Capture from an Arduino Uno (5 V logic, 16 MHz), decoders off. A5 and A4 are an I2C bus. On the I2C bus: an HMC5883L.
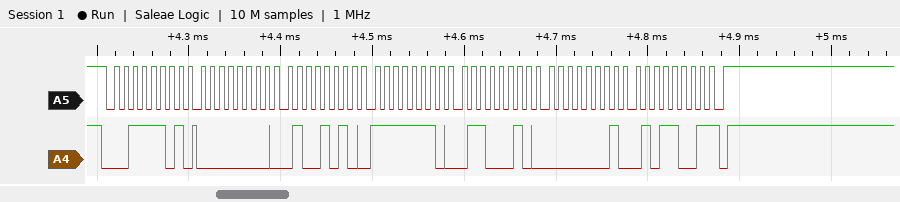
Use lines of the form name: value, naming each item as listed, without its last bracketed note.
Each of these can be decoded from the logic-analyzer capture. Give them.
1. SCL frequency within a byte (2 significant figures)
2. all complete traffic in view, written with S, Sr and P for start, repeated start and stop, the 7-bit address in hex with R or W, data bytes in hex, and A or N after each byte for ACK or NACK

SCL frequency within a byte: 100 kHz
all complete traffic in view, written with S, Sr and P for start, repeated start and stop, the 7-bit address in hex with R or W, data bytes in hex, and A or N after each byte for ACK or NACK: S 1ER A 00 A 4A A FE A 62 A 01 A 59 N P
